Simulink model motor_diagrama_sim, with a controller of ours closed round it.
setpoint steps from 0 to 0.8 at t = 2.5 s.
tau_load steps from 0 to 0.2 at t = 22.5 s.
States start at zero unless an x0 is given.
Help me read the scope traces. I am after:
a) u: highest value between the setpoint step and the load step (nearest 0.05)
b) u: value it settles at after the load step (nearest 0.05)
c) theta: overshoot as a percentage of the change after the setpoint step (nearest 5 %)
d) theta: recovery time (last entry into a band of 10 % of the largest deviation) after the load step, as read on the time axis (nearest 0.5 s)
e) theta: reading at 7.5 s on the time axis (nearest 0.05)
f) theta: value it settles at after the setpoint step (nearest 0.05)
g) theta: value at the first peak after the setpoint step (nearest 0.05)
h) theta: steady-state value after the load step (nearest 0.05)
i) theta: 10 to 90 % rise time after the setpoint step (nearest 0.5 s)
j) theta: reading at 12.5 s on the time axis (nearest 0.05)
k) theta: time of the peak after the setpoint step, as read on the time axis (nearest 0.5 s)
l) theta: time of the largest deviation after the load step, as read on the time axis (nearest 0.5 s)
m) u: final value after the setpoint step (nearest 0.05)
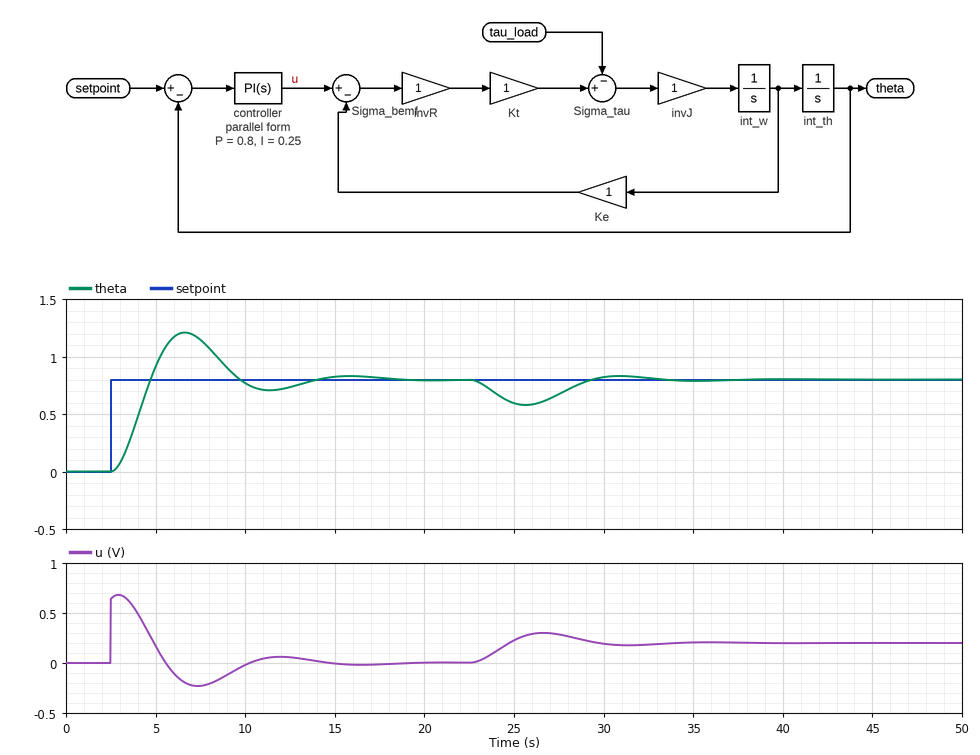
0.70
0.20
50 %
32.0 s
1.15
0.80
1.20
0.80
1.5 s
0.75
6.5 s
25.5 s
0.00
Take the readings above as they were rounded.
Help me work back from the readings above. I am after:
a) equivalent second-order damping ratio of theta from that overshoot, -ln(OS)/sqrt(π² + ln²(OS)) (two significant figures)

0.22
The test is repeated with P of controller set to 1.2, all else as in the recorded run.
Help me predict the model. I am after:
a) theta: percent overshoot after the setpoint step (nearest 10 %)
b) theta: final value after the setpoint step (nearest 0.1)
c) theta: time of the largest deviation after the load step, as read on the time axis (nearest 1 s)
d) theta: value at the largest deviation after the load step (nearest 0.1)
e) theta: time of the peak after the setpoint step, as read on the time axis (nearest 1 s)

40 %
0.8
25 s
0.6
6 s
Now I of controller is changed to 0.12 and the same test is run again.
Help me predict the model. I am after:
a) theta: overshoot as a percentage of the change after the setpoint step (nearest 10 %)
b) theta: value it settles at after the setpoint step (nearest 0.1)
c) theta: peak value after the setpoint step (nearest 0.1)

30 %
0.8
1.1
